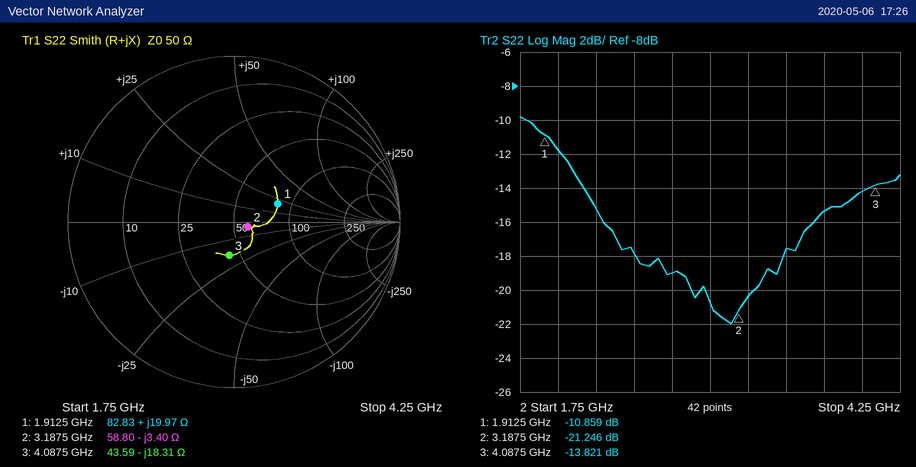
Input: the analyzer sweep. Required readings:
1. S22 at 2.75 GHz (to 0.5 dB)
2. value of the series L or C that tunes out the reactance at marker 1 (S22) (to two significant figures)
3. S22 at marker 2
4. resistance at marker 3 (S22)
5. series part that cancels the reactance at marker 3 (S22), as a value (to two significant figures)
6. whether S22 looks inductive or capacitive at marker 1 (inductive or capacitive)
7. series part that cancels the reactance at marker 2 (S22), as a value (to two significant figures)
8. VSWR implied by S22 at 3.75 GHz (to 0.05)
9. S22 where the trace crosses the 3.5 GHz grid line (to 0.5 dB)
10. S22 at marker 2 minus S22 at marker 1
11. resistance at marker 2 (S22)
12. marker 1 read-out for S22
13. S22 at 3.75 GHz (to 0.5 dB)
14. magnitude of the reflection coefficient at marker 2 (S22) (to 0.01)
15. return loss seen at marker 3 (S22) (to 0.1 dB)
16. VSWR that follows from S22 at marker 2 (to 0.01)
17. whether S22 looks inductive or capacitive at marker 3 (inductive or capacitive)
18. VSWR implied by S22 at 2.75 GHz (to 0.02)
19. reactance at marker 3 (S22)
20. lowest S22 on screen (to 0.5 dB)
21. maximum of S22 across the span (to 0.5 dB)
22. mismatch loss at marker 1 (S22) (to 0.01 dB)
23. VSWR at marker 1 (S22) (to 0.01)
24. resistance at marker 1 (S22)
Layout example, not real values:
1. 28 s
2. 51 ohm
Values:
1. -19.0 dB
2. 4.2 pF
3. -21.246 dB
4. 43.59 Ω
5. 710 pH
6. inductive
7. 170 pH
8. 1.40
9. -17.5 dB
10. -10.387 dB
11. 58.80 Ω
12. -10.859 dB
13. -15.5 dB
14. 0.09
15. 13.8 dB
16. 1.19
17. capacitive
18. 1.26
19. -18.31 Ω
20. -22.0 dB
21. -10.0 dB
22. 0.37 dB
23. 1.80
24. 82.83 Ω
